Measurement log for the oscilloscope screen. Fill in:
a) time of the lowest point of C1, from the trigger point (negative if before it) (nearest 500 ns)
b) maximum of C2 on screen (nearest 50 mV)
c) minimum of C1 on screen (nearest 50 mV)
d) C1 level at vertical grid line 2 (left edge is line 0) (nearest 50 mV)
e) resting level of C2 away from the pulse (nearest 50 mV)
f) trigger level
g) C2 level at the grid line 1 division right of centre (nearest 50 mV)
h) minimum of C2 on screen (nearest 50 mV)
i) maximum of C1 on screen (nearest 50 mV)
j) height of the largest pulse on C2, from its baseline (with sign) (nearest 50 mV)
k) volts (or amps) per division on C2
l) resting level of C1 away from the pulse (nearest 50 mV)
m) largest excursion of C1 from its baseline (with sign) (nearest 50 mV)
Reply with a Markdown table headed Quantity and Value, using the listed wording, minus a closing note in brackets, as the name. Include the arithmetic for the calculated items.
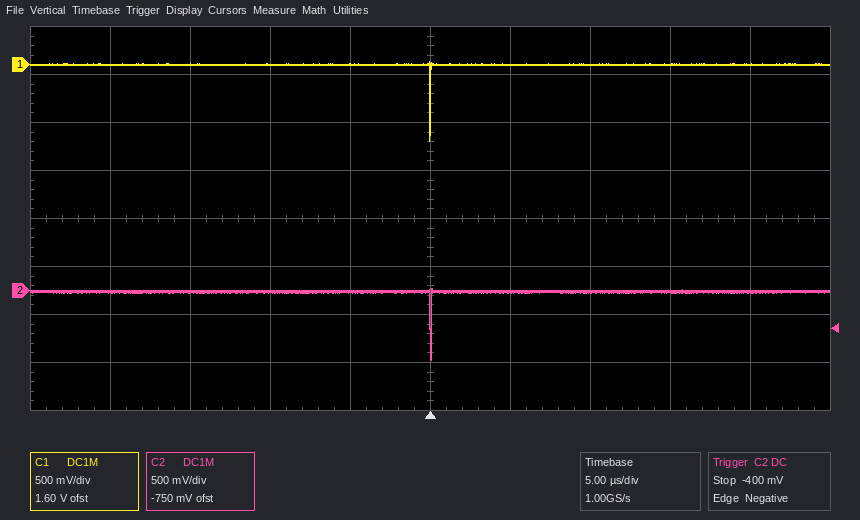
| Quantity | Value |
|---|---|
| time of the lowest point of C1, from the trigger point (negative if before it) | 0.0 µs |
| maximum of C2 on screen | 0 mV |
| minimum of C1 on screen | -800 mV |
| C1 level at vertical grid line 2 (left edge is line 0) | 0 mV |
| resting level of C2 away from the pulse | 0 mV |
| trigger level | -400 mV |
| C2 level at the grid line 1 division right of centre | 0 mV |
| minimum of C2 on screen | -700 mV |
| maximum of C1 on screen | 50 mV |
| height of the largest pulse on C2, from its baseline (with sign) | -700 mV − (0 mV) = -700 mV |
| volts (or amps) per division on C2 | 500 mV |
| resting level of C1 away from the pulse | 0 mV |
| largest excursion of C1 from its baseline (with sign) | -800 mV − (0 mV) = -800 mV |
